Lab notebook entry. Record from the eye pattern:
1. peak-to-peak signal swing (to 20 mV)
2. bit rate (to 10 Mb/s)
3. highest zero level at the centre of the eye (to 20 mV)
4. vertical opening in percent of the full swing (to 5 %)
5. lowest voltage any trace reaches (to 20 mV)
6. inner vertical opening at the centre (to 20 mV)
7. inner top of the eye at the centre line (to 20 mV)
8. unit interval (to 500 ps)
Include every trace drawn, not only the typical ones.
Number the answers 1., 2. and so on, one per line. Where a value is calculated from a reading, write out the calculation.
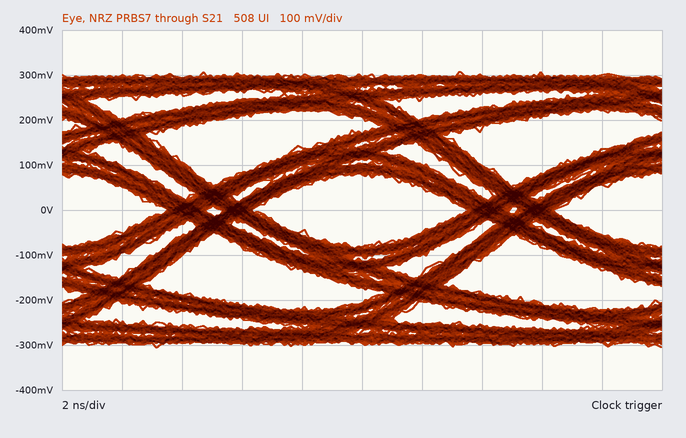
1. 620 mV
2. 100 Mb/s
3. -80 mV
4. 160 mV / 620 mV ≈ 25.8 %, so 25 % to the nearest 5 %
5. -300 mV
6. 160 mV
7. 80 mV
8. 10.0 ns
